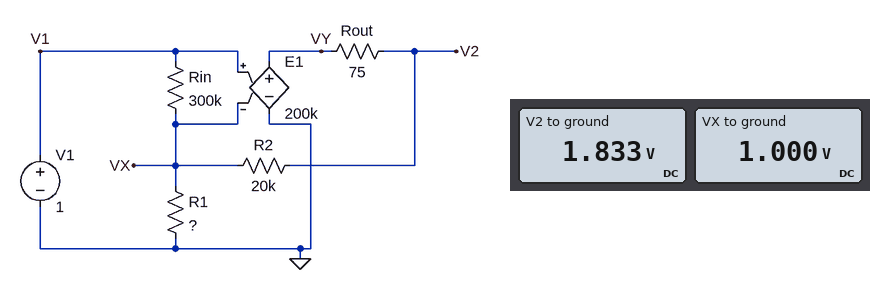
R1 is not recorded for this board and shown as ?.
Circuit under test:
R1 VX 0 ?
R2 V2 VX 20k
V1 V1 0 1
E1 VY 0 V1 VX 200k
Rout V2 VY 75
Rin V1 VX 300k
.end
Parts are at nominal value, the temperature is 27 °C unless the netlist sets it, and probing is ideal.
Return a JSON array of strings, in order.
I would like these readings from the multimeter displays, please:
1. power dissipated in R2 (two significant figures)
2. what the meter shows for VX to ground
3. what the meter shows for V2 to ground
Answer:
["35 µW", "1.000 V", "1.833 V"]
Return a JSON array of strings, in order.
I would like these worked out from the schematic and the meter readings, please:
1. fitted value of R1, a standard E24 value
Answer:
["24 kΩ"]
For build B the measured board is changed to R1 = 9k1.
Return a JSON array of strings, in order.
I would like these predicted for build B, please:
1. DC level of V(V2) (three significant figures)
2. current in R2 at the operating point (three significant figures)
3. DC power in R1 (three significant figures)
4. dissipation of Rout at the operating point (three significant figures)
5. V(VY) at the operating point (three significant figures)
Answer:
["3.20 V", "110 µA", "110 µW", "906 nW", "3.21 V"]
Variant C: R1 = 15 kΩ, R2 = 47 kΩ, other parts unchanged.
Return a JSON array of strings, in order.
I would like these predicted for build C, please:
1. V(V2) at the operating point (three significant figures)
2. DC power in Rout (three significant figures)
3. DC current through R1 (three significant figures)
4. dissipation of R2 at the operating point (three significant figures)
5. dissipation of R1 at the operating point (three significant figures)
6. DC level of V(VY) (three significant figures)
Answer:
["4.13 V", "333 nW", "66.7 µA", "209 µW", "66.7 µW", "4.14 V"]
